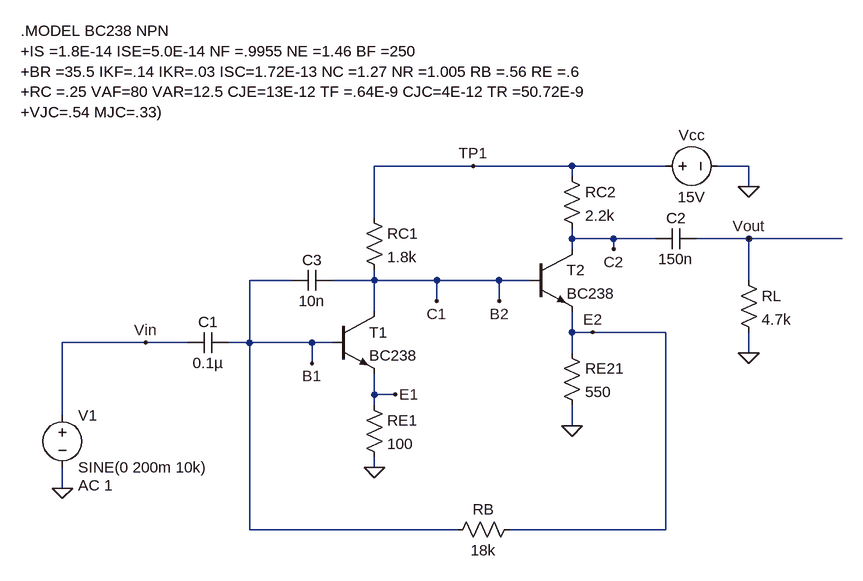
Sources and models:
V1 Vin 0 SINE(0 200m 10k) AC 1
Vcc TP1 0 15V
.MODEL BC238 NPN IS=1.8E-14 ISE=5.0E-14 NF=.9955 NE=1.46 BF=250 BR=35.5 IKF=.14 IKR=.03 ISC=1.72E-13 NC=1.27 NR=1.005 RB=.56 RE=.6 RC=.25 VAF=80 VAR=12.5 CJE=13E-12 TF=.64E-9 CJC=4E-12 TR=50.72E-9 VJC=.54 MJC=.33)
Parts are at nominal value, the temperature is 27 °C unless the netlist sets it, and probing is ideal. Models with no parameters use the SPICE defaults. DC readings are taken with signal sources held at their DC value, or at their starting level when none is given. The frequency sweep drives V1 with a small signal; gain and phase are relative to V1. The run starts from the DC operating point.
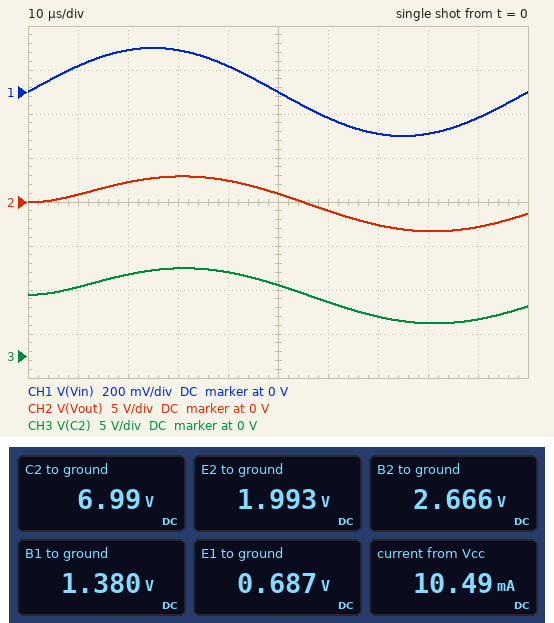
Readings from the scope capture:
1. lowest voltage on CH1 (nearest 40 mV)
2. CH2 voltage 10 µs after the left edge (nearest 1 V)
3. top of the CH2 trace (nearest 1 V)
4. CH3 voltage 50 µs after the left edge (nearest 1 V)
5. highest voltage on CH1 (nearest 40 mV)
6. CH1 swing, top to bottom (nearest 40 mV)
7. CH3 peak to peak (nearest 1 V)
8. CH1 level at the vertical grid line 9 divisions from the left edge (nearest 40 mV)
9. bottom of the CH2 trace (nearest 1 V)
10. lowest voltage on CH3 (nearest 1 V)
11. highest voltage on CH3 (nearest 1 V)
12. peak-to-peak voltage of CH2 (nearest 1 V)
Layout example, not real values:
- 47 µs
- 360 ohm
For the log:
- -200 mV
- 1 V
- 3 V
- 8 V
- 200 mV
- 400 mV
- 6 V
- -120 mV
- -3 V
- 4 V
- 10 V
- 6 V
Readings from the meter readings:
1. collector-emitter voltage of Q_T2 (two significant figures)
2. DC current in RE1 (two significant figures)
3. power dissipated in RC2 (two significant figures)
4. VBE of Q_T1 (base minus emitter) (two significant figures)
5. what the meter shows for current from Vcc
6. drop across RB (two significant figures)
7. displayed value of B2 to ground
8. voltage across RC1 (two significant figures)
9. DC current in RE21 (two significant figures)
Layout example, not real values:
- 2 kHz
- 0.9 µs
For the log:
- 5.0 V
- 6.9 mA
- 29 mW
- 690 mV
- 10.49 mA
- 610 mV
- 2.666 V
- 12 V
- 3.6 mA
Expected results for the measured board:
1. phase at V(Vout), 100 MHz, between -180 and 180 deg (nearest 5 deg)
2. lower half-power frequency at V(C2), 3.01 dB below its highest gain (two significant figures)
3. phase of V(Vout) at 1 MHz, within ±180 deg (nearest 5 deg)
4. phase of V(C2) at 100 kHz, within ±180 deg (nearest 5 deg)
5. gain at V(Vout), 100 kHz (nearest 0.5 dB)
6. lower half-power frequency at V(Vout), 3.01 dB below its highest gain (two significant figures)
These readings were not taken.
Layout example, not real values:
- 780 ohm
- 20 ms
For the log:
- 65 deg
- 530 Hz
- -170 deg
- -110 deg
- 13.5 dB
- 610 Hz
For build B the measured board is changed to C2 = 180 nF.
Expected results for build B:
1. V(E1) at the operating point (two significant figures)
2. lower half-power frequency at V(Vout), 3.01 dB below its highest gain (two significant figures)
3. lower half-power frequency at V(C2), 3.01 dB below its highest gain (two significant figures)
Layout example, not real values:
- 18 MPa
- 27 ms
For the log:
- 690 mV
- 600 Hz
- 540 Hz
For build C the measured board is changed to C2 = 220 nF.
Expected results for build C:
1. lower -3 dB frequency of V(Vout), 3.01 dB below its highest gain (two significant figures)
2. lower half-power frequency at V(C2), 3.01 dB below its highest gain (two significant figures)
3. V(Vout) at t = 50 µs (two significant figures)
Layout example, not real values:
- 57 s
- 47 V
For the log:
- 590 Hz
- 550 Hz
- 970 mV
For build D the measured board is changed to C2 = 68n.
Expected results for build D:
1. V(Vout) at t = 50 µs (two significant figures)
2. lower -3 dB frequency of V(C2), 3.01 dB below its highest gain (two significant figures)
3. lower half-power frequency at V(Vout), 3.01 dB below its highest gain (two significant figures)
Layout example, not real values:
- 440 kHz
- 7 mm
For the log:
- 840 mV
- 420 Hz
- 710 Hz
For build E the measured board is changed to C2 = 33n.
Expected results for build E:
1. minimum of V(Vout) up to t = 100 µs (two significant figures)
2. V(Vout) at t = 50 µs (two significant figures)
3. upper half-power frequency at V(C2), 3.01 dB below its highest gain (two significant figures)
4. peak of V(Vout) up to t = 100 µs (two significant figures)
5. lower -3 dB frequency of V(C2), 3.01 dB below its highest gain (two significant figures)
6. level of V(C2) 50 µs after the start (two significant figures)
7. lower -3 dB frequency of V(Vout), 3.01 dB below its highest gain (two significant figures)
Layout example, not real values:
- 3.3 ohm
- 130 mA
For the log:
- -3.4 V
- 660 mV
- 24 kHz
- 2.8 V
- 370 Hz
- 8.2 V
- 950 Hz
